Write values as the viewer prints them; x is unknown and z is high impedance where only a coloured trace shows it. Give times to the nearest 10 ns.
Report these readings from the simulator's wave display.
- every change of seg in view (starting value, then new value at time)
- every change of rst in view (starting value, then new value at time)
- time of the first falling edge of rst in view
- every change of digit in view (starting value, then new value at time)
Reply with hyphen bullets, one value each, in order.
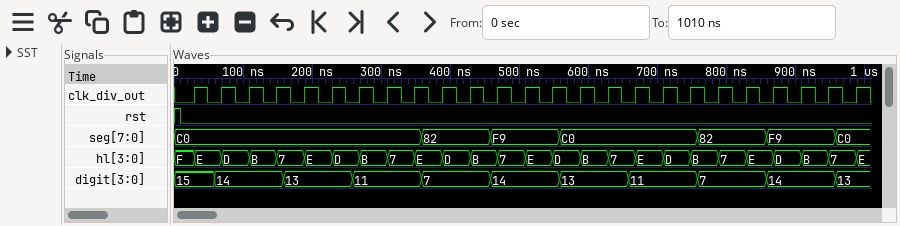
- C0, 82 at 360 ns, F9 at 460 ns, C0 at 560 ns, 82 at 760 ns, F9 at 860 ns, C0 at 960 ns
- 1, 0 at 10 ns
- 10 ns
- 15, 14 at 60 ns, 13 at 160 ns, 11 at 260 ns, 7 at 360 ns, 14 at 460 ns, 13 at 560 ns, 11 at 660 ns, 7 at 760 ns, 14 at 860 ns, 13 at 960 ns
